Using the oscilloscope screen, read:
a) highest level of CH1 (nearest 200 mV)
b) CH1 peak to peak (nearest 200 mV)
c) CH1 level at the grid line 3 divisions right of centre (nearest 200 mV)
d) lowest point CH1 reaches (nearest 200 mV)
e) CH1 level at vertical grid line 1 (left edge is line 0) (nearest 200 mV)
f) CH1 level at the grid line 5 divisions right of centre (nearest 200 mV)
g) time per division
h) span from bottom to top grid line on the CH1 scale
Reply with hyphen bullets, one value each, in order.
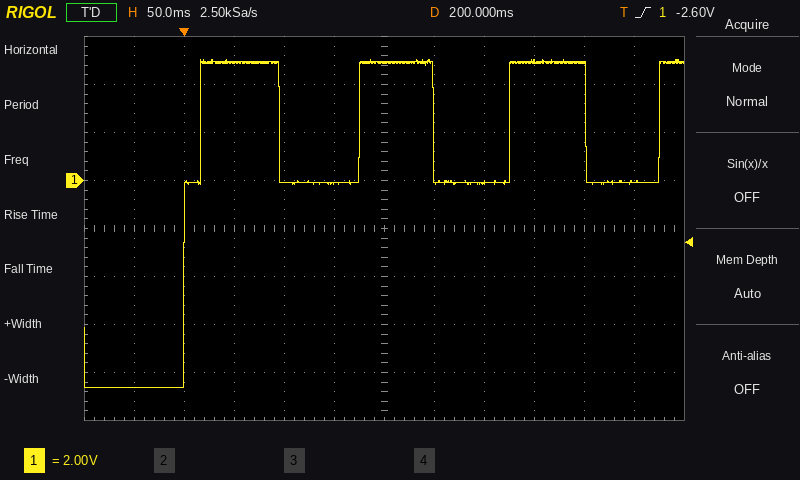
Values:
- 5.0 V
- 13.6 V
- 5.0 V
- -8.6 V
- -8.6 V
- 0.0 V
- 50 ms
- 16 V
